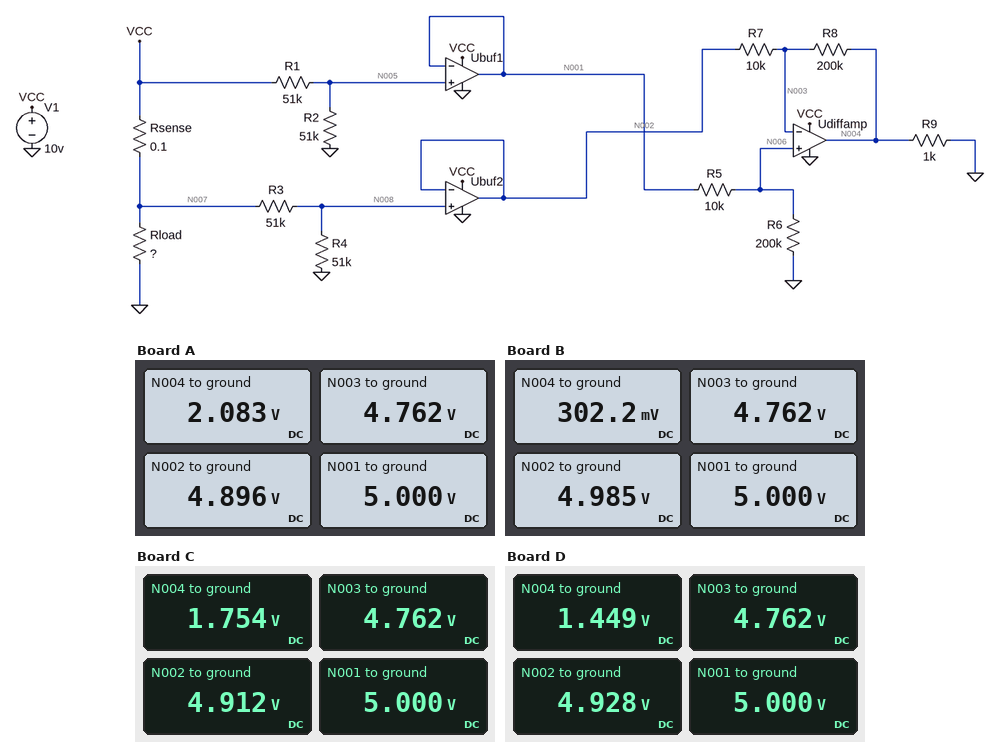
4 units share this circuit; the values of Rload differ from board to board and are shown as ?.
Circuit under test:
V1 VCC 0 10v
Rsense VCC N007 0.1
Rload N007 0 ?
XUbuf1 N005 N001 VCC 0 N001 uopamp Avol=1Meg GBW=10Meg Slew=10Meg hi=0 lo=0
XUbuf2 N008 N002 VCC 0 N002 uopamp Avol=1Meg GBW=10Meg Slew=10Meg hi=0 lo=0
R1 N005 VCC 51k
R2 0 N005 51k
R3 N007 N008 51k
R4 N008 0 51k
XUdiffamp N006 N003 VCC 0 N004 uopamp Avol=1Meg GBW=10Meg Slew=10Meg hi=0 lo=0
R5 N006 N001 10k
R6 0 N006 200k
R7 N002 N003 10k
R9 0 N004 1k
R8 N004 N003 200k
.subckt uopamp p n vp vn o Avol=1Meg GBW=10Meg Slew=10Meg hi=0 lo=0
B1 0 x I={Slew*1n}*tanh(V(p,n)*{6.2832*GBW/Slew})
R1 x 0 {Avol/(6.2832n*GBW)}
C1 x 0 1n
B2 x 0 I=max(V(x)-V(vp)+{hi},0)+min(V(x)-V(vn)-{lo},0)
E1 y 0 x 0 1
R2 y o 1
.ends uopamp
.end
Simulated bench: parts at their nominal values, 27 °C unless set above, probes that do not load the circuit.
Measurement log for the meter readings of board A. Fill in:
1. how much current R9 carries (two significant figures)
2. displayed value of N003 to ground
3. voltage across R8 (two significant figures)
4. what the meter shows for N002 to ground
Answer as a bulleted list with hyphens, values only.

- 2.1 mA
- 4.762 V
- 2.7 V
- 4.896 V
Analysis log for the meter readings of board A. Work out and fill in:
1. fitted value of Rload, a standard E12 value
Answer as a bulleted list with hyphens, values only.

- 4.7 Ω
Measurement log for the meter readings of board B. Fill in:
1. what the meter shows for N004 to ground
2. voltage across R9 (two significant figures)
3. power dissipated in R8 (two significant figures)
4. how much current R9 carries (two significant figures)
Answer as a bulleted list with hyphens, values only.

- 302.2 mV
- 300 mV
- 99 µW
- 300 µA
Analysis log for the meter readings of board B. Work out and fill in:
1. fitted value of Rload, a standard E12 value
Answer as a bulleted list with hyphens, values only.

- 33 Ω
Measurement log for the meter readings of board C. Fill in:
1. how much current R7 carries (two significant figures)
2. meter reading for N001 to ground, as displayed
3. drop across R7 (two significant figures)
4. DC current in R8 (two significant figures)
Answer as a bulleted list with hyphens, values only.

- 15 µA
- 5.000 V
- 150 mV
- 15 µA
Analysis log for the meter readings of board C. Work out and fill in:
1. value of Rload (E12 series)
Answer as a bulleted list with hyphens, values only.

- 5.6 Ω
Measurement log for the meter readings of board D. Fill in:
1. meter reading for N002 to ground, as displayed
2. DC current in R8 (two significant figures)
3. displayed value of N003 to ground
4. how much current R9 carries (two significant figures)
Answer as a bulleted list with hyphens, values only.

- 4.928 V
- 17 µA
- 4.762 V
- 1.4 mA
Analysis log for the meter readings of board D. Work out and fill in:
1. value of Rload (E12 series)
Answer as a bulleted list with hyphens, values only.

- 6.8 Ω
